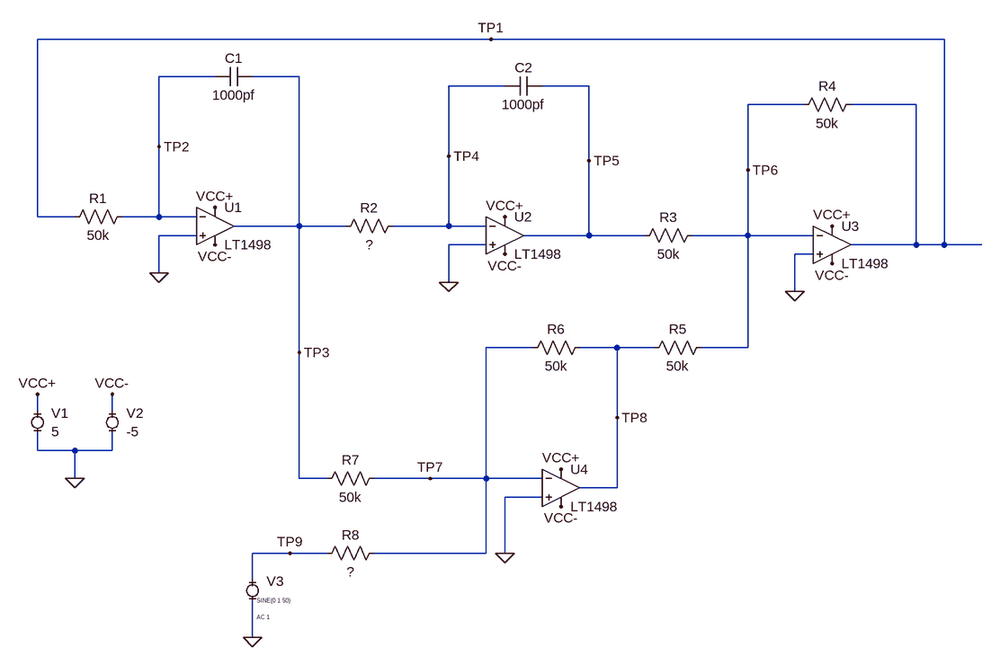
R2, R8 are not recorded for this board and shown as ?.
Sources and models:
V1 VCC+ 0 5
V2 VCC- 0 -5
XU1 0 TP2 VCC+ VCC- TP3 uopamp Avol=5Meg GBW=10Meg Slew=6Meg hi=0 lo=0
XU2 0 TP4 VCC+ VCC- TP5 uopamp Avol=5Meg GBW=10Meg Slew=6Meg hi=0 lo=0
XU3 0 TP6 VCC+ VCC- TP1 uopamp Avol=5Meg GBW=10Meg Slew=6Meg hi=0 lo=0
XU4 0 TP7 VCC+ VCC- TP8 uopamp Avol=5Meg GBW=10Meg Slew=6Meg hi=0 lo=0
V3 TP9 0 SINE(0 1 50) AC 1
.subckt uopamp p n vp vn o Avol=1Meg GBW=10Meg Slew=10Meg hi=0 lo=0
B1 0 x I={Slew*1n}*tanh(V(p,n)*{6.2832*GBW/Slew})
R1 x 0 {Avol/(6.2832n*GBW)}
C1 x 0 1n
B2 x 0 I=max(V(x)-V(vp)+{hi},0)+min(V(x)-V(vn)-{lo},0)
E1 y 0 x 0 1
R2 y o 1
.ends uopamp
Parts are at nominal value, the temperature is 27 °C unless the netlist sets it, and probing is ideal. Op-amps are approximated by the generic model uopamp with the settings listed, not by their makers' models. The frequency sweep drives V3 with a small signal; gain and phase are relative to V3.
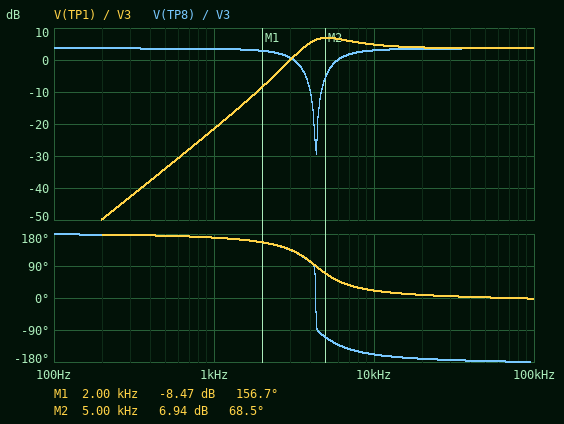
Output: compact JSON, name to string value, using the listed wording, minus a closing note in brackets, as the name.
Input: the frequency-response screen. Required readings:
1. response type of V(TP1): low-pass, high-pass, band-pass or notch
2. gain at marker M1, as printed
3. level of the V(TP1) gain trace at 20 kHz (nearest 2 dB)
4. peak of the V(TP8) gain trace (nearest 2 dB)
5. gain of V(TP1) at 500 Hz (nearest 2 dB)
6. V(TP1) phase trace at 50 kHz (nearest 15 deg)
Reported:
{"response type of V(TP1): low-pass, high-pass, band-pass or notch": "high-pass", "gain at marker M1, as printed": "-8.47 dB", "level of the V(TP1) gain trace at 20 kHz": "4 dB", "peak of the V(TP8) gain trace": "4 dB", "gain of V(TP1) at 500 Hz": "-34 dB", "V(TP1) phase trace at 50 kHz": "0 deg"}
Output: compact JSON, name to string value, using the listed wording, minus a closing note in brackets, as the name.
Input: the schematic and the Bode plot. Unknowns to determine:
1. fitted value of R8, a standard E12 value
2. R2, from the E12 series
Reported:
{"fitted value of R8, a standard E12 value": "33 kΩ", "R2, from the E12 series": "27 kΩ"}
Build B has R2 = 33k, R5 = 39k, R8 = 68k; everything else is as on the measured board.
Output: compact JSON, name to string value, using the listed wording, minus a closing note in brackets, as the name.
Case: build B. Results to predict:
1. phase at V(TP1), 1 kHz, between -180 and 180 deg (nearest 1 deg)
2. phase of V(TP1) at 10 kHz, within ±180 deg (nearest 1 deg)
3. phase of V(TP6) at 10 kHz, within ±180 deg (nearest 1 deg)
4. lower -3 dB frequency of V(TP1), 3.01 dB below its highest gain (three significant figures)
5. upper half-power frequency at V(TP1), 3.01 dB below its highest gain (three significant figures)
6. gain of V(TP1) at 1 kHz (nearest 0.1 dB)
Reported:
{"phase at V(TP1), 1 kHz, between -180 and 180 deg": "164 deg", "phase of V(TP1) at 10 kHz, within ±180 deg": "25 deg", "phase of V(TP6) at 10 kHz, within ±180 deg": "-65 deg", "lower -3 dB frequency of V(TP1), 3.01 dB below its highest gain": "3.38 kHz", "upper half-power frequency at V(TP1), 3.01 dB below its highest gain": "1.68 MHz", "gain of V(TP1) at 1 kHz": "-24.0 dB"}
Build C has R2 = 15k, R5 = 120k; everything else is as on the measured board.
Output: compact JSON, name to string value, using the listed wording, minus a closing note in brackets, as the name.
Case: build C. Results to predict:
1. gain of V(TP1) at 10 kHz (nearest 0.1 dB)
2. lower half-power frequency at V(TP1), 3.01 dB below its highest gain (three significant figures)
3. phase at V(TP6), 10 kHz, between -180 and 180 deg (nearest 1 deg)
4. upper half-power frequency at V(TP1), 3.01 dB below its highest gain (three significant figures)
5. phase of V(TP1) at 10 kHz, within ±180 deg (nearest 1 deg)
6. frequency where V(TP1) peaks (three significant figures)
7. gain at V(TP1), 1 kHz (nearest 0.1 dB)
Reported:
{"gain of V(TP1) at 10 kHz": "-0.6 dB", "lower half-power frequency at V(TP1), 3.01 dB below its highest gain": "5.31 kHz", "phase at V(TP6), 10 kHz, between -180 and 180 deg": "-79 deg", "upper half-power frequency at V(TP1), 3.01 dB below its highest gain": "6.71 kHz", "phase of V(TP1) at 10 kHz, within ±180 deg": "11 deg", "frequency where V(TP1) peaks": "5.89 kHz", "gain at V(TP1), 1 kHz": "-34.3 dB"}
